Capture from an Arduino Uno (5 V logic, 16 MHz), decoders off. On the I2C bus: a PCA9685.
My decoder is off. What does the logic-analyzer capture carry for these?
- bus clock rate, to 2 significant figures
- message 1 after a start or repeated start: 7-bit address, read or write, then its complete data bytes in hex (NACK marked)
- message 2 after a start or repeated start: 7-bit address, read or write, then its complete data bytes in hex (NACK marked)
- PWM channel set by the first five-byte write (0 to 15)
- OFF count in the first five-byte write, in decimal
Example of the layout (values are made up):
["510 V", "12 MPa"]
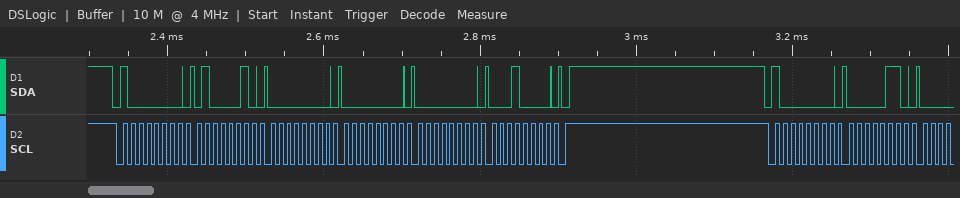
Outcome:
["100 kHz", "0x40 write: 42 00 00 00 10", "0x40 write: 06", "15", "4096"]
